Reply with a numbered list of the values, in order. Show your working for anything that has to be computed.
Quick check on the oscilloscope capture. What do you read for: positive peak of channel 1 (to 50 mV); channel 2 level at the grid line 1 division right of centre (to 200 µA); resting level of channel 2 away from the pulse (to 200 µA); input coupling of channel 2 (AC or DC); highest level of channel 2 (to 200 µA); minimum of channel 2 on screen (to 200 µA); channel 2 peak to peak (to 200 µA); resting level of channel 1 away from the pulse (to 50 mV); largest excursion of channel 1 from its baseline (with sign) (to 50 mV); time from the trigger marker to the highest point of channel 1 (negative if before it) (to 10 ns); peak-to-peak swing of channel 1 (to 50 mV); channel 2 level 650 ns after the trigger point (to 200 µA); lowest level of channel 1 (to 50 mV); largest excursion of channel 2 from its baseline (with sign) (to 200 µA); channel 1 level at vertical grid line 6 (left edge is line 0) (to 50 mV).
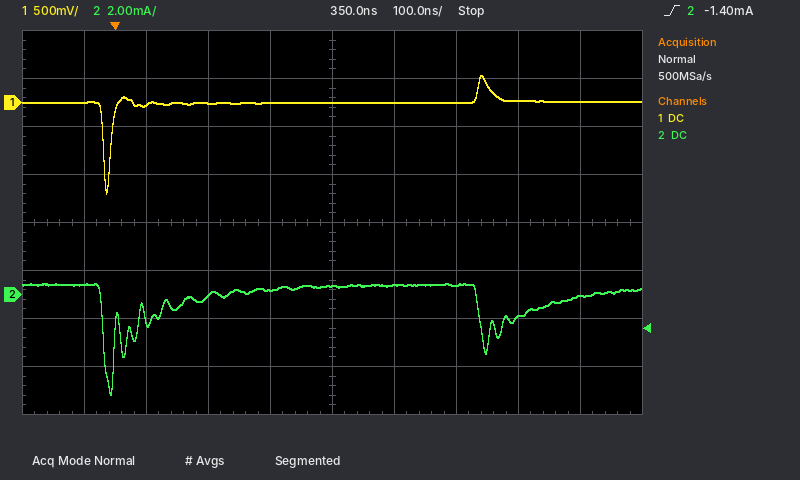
1. 300 mV
2. 400 µA
3. 400 µA
4. DC
5. 400 µA
6. -4.2 mA
7. 400 µA − (-4.2 mA) = 4.6 mA
8. 0 mV
9. -950 mV − (0 mV) = -950 mV
10. +590 ns
11. 300 mV − (-950 mV) = 1.25 V
12. -1.0 mA
13. -950 mV
14. -4.2 mA − (400 µA) = -4.6 mA
15. 0 mV
